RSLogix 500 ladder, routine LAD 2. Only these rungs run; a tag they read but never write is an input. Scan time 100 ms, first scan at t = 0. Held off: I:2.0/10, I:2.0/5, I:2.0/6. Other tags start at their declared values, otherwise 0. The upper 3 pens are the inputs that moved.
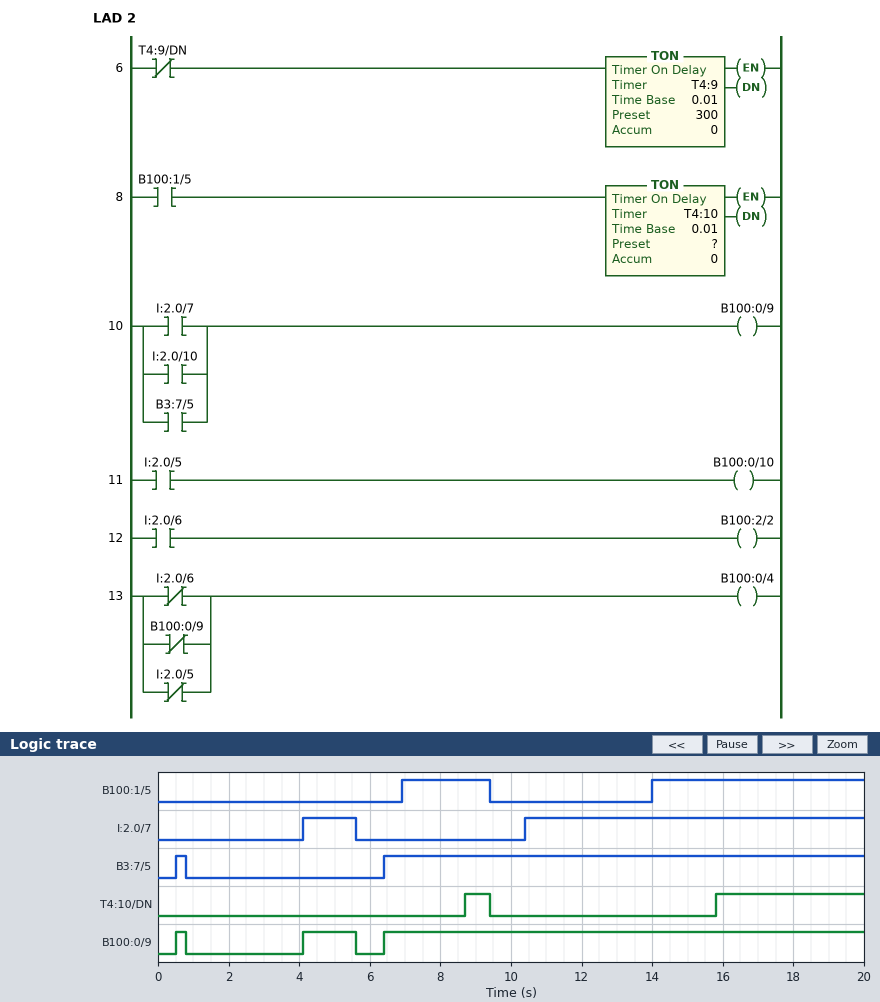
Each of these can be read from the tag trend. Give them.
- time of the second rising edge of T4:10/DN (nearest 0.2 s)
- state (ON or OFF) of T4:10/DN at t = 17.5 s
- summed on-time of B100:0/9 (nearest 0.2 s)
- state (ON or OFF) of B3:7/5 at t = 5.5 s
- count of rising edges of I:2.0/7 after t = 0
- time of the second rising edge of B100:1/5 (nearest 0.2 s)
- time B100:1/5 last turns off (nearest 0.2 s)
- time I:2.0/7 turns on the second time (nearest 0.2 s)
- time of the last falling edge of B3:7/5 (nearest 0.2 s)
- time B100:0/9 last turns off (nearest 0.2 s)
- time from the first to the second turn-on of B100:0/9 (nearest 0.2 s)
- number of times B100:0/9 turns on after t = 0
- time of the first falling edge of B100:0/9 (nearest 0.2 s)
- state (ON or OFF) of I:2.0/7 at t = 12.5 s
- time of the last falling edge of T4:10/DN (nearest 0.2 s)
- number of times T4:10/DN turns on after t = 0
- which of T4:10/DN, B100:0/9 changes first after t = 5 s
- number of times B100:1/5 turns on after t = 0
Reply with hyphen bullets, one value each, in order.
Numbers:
- 15.8 s
- ON
- 15.4 s
- OFF
- 2
- 14.0 s
- 9.4 s
- 10.4 s
- 0.8 s
- 5.6 s
- 3.6 s
- 3
- 0.8 s
- ON
- 9.4 s
- 2
- B100:0/9
- 2
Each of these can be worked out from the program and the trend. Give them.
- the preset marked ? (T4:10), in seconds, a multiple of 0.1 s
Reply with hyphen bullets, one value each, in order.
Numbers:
- 1.8 s
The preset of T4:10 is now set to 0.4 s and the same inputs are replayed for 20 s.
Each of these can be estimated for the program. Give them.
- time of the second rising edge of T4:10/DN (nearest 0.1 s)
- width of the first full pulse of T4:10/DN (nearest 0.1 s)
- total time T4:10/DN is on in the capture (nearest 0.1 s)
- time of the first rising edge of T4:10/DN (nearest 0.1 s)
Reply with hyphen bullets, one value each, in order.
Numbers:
- 14.4 s
- 2.1 s
- 7.7 s
- 7.3 s
